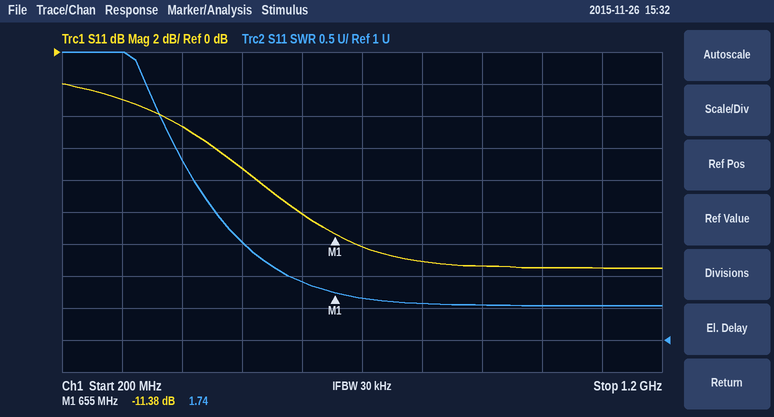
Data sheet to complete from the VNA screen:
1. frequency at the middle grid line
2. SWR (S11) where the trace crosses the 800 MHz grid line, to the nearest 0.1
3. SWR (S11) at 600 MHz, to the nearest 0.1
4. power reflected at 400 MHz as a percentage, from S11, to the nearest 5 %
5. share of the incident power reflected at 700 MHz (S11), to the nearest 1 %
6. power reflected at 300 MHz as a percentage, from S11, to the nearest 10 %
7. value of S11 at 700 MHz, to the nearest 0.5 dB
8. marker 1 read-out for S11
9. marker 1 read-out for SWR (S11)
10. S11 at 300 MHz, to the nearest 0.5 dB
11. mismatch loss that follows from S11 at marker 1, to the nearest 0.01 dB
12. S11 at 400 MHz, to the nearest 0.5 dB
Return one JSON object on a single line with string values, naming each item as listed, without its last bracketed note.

{"frequency at the middle grid line": "700 MHz", "SWR (S11) where the trace crosses the 800 MHz grid line, to the nearest 0.1": "1.6", "SWR (S11) at 600 MHz, to the nearest 0.1": "1.9", "power reflected at 400 MHz as a percentage, from S11, to the nearest 5 %": "35 %", "share of the incident power reflected at 700 MHz (S11), to the nearest 1 %": "6 %", "power reflected at 300 MHz as a percentage, from S11, to the nearest 10 %": "50 %", "value of S11 at 700 MHz, to the nearest 0.5 dB": "-12.0 dB", "marker 1 read-out for S11": "-11.38 dB", "marker 1 read-out for SWR": "1.74", "S11 at 300 MHz, to the nearest 0.5 dB": "-3.0 dB", "mismatch loss that follows from S11 at marker 1, to the nearest 0.01 dB": "0.33 dB", "S11 at 400 MHz, to the nearest 0.5 dB": "-4.5 dB"}
